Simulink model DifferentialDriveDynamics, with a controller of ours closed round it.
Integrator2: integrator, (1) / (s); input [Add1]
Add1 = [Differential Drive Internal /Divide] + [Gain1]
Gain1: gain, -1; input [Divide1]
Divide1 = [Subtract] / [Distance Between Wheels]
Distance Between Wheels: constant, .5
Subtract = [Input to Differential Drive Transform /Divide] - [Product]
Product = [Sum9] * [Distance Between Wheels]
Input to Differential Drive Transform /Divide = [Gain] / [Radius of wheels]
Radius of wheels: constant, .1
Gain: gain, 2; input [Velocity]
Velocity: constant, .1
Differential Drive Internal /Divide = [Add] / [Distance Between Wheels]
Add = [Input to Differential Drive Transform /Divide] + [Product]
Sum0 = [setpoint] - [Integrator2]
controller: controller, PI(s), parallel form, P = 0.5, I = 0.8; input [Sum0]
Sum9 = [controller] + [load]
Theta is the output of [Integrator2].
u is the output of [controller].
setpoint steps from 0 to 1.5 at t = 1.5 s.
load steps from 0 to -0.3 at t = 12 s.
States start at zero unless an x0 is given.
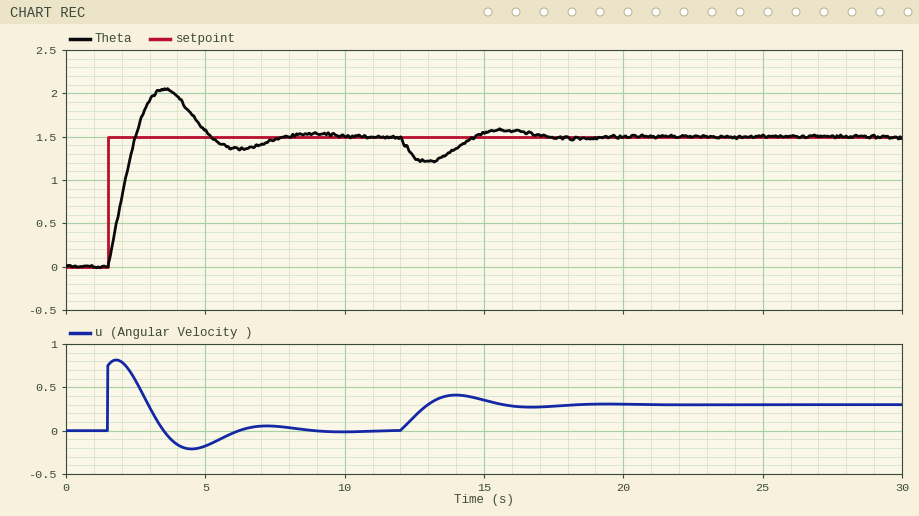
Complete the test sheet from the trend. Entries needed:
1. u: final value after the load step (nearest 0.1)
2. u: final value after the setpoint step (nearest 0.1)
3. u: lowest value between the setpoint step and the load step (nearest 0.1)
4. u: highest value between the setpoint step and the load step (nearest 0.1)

0.3
0.0
-0.2
0.8
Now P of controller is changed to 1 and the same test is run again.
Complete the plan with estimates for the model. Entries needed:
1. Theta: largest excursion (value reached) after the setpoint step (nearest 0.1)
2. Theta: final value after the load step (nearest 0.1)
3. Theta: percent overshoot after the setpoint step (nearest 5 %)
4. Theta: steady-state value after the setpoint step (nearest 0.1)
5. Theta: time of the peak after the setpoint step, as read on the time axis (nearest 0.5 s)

1.8
1.5
20 %
1.5
3.0 s
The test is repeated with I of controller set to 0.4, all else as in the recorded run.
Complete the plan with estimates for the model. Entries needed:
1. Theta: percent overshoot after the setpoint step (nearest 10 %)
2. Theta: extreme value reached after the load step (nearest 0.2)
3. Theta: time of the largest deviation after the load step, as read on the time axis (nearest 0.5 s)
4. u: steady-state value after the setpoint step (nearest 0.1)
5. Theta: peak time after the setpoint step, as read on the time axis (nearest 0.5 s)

30 %
1.2
13.5 s
0.0
4.0 s
